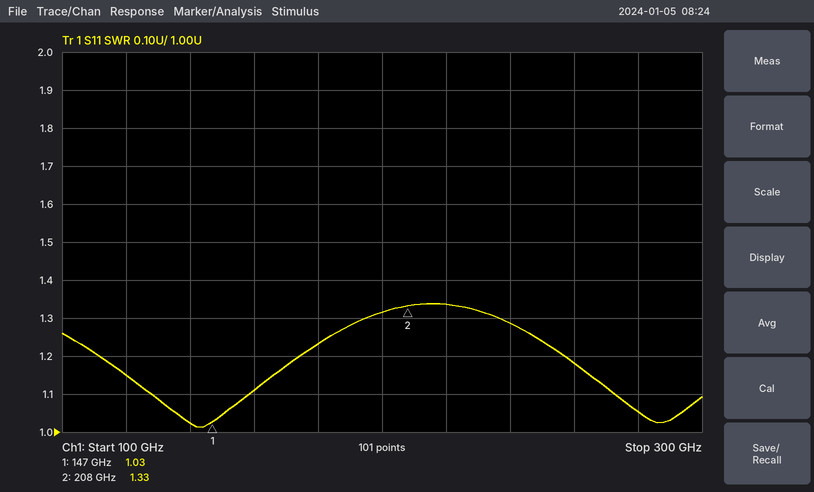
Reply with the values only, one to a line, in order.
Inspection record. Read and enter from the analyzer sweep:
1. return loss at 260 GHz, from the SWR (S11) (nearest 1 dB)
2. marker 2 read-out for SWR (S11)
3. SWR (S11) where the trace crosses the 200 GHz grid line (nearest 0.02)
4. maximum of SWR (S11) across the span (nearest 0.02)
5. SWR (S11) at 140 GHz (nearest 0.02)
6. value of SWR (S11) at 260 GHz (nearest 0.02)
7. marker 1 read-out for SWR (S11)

22 dB
1.33
1.32
1.34
1.02
1.18
1.03
